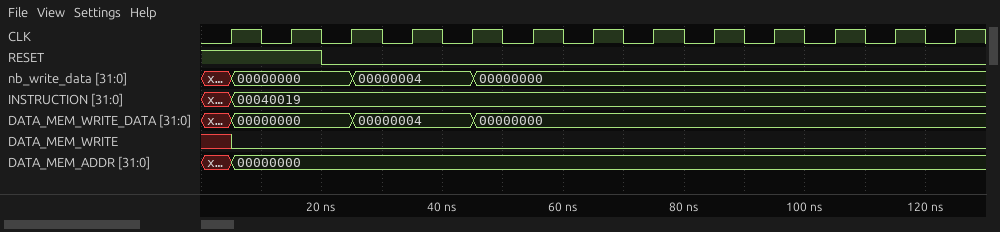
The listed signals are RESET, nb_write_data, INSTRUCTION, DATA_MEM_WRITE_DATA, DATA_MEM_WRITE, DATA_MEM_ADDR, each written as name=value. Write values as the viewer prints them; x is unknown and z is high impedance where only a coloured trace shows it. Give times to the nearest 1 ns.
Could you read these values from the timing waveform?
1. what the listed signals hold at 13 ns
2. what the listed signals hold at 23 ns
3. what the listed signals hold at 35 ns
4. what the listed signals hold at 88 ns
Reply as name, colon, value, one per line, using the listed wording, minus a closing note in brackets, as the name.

what the listed signals hold at 13 ns: RESET=1, nb_write_data=00000000, INSTRUCTION=00040019, DATA_MEM_WRITE_DATA=00000000, DATA_MEM_WRITE=0, DATA_MEM_ADDR=00000000
what the listed signals hold at 23 ns: RESET=0, nb_write_data=00000000, INSTRUCTION=00040019, DATA_MEM_WRITE_DATA=00000000, DATA_MEM_WRITE=0, DATA_MEM_ADDR=00000000
what the listed signals hold at 35 ns: RESET=0, nb_write_data=00000004, INSTRUCTION=00040019, DATA_MEM_WRITE_DATA=00000004, DATA_MEM_WRITE=0, DATA_MEM_ADDR=00000000
what the listed signals hold at 88 ns: RESET=0, nb_write_data=00000000, INSTRUCTION=00040019, DATA_MEM_WRITE_DATA=00000000, DATA_MEM_WRITE=0, DATA_MEM_ADDR=00000000
